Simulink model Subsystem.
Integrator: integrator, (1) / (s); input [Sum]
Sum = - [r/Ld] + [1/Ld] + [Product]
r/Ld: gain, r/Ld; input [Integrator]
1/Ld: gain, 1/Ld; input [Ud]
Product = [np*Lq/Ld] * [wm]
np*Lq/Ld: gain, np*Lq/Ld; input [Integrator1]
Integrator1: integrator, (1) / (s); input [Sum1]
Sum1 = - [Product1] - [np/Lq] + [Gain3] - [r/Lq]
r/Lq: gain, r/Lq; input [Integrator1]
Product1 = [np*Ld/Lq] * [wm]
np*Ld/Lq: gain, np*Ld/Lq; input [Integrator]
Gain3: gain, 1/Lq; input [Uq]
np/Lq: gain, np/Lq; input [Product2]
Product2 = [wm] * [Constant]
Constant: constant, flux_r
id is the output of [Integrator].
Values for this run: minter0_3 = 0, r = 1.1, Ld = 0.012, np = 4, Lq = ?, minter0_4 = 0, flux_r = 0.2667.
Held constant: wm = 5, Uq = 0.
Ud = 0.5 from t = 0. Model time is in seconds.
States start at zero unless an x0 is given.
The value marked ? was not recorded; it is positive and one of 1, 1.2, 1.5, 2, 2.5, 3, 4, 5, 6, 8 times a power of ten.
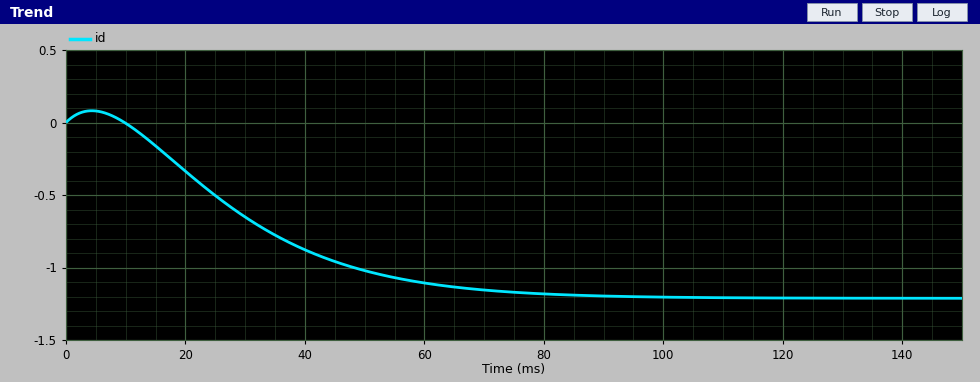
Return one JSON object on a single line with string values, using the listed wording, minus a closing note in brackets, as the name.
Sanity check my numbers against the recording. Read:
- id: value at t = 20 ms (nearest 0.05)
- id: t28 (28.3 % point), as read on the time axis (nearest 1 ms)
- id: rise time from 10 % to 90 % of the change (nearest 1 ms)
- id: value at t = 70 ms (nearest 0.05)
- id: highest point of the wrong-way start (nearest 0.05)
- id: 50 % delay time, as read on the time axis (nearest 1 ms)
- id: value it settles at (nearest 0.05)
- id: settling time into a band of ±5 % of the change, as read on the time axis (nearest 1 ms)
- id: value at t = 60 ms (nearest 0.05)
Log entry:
{"id: value at t = 20 ms": "-0.35", "id: t28 (28.3 % point), as read on the time axis": "20 ms", "id: rise time from 10 % to 90 % of the change": "44 ms", "id: value at t = 70 ms": "-1.15", "id: highest point of the wrong-way start": "0.10", "id: 50 % delay time, as read on the time axis": "28 ms", "id: value it settles at": "-1.20", "id: settling time into a band of ±5 % of the change, as read on the time axis": "69 ms", "id: value at t = 60 ms": "-1.10"}
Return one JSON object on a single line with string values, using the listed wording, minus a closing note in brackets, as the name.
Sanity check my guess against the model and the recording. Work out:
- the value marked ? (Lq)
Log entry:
{"the value marked ?": "0.02"}
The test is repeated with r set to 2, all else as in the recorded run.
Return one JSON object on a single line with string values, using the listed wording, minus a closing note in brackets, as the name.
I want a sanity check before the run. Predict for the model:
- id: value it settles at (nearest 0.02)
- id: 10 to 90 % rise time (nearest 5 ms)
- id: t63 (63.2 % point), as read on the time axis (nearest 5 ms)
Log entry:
{"id: value it settles at": "-0.28", "id: 10 to 90 % rise time": "25 ms", "id: t63 (63.2 % point), as read on the time axis": "25 ms"}
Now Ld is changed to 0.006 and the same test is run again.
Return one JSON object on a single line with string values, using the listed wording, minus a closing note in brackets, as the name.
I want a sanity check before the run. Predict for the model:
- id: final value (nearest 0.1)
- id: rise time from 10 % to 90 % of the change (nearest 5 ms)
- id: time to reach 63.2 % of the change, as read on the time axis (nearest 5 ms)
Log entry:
{"id: final value": "-1.3", "id: rise time from 10 % to 90 % of the change": "40 ms", "id: time to reach 63.2 % of the change, as read on the time axis": "30 ms"}
